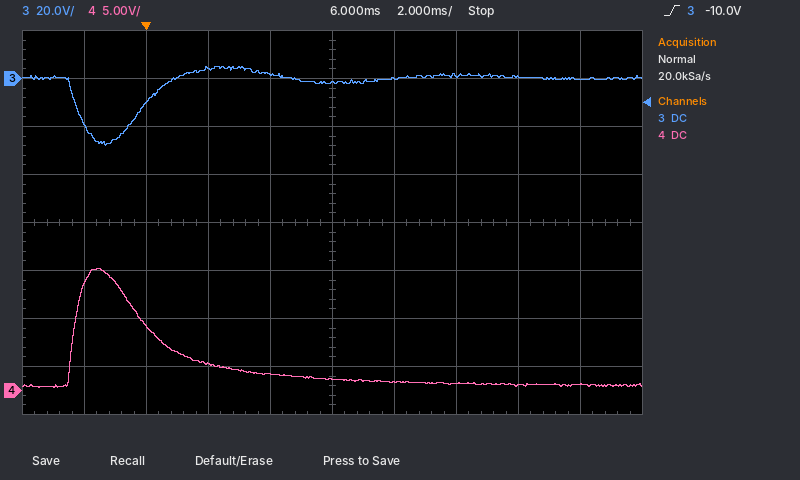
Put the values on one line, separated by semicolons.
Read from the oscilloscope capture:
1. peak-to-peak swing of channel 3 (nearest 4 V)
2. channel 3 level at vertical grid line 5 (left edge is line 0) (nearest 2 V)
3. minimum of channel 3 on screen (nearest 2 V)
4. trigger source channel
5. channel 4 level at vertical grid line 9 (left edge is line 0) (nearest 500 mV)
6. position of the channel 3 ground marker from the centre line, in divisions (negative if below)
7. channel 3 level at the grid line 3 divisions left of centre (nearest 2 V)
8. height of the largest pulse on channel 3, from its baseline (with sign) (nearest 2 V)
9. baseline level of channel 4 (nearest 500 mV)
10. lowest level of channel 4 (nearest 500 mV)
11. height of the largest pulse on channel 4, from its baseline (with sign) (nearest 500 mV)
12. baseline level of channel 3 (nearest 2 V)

32 V; -2 V; -28 V; channel 3; 500 mV; +3.0 div; -10 V; -28 V; 500 mV; 500 mV; +12.0 V; 0 V
